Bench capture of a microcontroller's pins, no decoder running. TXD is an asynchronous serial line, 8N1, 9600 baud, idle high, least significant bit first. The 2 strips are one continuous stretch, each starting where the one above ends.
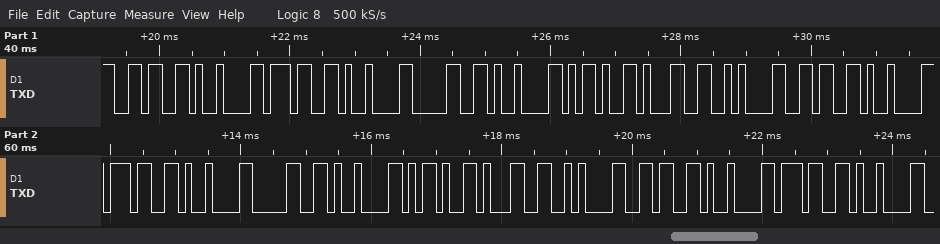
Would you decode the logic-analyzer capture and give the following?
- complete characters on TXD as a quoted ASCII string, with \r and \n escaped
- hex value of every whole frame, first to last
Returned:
"6\t7\t0\t-1\n6\t7\t0\t-1\n6\t7\t"
36 09 37 09 30 09 2D 31 0A 36 09 37 09 30 09 2D 31 0A 36 09 37 09
